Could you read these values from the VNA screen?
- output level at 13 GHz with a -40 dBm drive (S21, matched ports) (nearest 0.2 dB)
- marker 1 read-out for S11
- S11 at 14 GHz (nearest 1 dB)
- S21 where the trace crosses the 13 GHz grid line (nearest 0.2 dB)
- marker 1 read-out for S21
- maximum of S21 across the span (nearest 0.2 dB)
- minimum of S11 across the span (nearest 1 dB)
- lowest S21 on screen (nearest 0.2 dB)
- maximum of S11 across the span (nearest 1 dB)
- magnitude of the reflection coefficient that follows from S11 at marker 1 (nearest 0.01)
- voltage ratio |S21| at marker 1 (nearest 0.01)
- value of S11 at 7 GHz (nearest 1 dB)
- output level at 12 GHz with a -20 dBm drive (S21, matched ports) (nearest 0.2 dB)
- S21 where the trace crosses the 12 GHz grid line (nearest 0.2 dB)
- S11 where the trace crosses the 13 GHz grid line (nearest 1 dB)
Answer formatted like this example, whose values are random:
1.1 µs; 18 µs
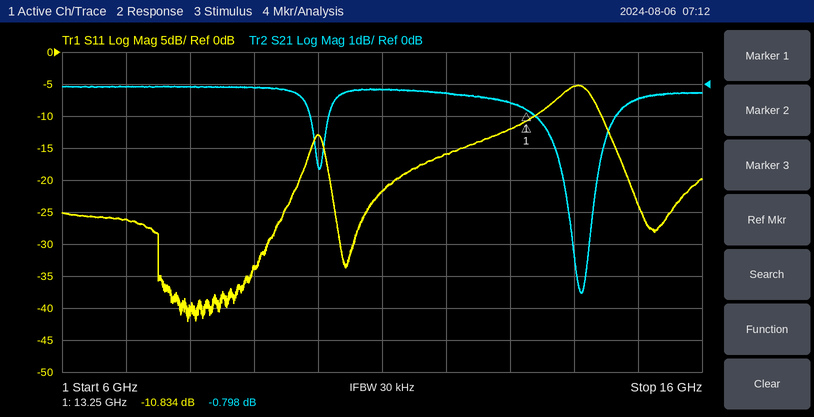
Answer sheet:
-40.6 dBm; -10.834 dB; -5 dB; -0.6 dB; -0.798 dB; 0.0 dB; -42 dB; -6.6 dB; -5 dB; 0.29; 0.91; -26 dB; -20.2 dBm; -0.2 dB; -12 dB
